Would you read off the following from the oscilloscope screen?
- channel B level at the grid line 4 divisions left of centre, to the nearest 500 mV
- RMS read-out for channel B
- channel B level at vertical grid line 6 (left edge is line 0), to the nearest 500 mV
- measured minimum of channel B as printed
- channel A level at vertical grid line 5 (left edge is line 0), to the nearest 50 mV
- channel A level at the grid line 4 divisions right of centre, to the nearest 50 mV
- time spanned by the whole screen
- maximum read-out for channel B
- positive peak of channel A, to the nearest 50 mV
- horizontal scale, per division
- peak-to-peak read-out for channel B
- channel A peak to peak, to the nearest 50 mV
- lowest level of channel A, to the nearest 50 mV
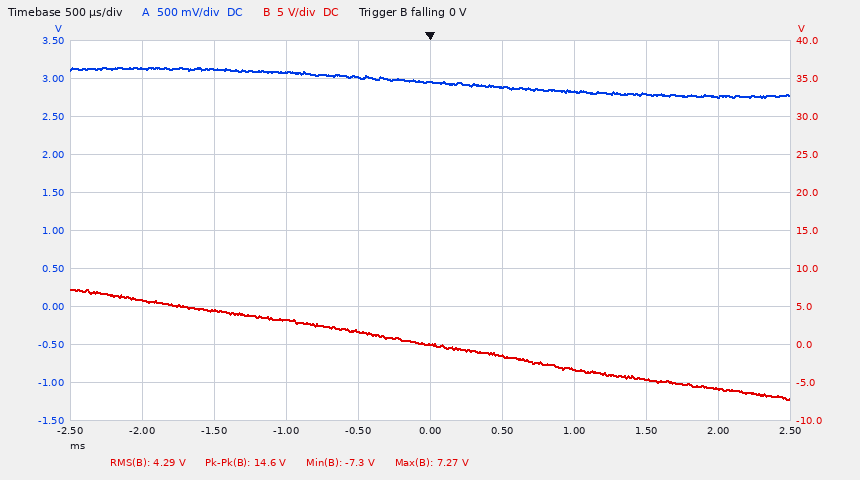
6.0 V
4.29 V
-1.5 V
-7.3 V
2.95 V
2.75 V
5 ms
7.27 V
3.15 V
500 µs
14.6 V
400 mV
2.75 V
